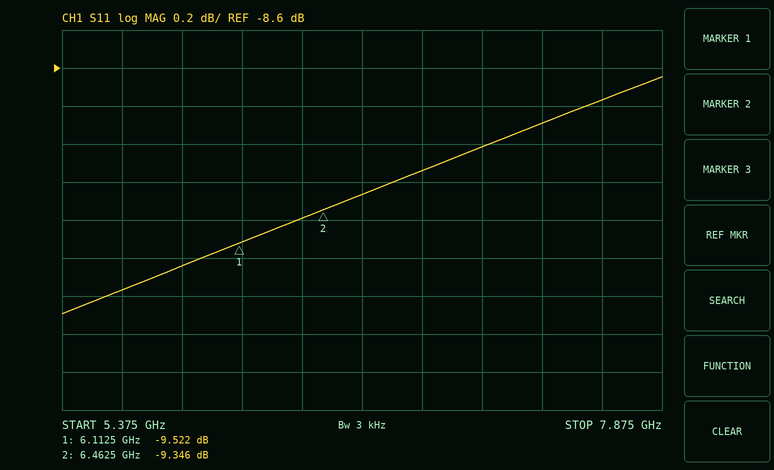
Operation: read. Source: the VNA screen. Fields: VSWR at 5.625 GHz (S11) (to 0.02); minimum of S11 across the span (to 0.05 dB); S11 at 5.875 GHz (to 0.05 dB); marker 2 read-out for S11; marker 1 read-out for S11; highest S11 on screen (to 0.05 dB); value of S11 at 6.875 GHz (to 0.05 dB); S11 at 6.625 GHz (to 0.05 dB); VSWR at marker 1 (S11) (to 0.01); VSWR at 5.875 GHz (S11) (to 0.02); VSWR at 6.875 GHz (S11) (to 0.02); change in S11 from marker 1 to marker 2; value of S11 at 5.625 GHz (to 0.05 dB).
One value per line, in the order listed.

1.96
-9.90 dB
-9.65 dB
-9.346 dB
-9.522 dB
-8.65 dB
-9.15 dB
-9.25 dB
2.00
1.98
2.08
0.176 dB
-9.75 dB
